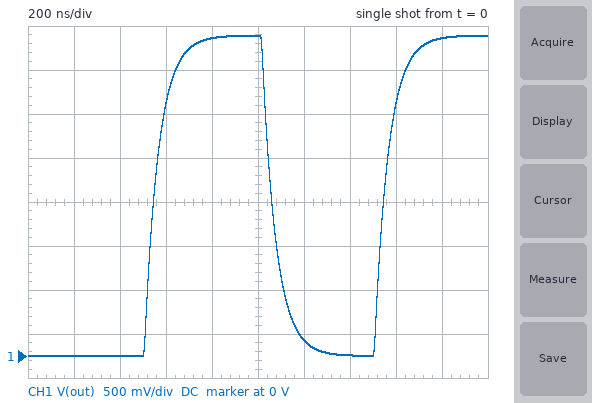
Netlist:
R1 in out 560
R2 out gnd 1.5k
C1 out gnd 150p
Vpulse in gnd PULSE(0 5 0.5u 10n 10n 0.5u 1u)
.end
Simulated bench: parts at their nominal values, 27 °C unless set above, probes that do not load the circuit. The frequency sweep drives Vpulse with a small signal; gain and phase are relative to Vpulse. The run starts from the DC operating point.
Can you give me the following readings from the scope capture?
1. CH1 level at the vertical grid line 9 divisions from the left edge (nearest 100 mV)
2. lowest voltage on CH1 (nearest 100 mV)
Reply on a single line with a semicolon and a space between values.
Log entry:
3.6 V; 0 V
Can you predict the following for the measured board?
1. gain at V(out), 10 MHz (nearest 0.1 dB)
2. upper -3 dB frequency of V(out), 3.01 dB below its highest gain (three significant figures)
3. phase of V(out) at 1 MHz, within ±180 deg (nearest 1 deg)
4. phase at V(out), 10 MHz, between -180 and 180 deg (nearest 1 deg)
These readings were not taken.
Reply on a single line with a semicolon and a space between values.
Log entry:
-14.7 dB; 2.60 MHz; -21 deg; -75 deg
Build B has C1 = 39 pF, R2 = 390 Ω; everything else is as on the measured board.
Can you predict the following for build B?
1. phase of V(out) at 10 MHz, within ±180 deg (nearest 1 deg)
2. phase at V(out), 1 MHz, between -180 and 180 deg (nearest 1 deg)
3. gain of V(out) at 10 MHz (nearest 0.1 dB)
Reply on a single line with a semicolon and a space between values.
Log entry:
-29 deg; -3 deg; -8.9 dB
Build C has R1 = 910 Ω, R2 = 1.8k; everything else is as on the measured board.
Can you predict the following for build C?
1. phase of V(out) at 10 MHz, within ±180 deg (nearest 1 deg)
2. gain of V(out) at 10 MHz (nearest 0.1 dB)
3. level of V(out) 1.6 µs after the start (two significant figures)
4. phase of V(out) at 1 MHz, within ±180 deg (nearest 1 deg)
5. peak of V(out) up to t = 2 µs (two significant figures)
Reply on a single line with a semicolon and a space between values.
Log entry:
-80 deg; -18.8 dB; 2.2 V; -30 deg; 3.3 V
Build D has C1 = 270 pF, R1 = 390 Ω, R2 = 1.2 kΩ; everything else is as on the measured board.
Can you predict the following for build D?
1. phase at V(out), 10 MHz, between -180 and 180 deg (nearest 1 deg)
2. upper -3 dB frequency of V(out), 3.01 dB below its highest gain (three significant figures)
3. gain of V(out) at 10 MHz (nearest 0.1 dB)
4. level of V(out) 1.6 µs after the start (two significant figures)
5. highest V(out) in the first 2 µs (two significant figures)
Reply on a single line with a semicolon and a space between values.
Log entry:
-79 deg; 2.00 MHz; -16.6 dB; 2.6 V; 3.8 V
